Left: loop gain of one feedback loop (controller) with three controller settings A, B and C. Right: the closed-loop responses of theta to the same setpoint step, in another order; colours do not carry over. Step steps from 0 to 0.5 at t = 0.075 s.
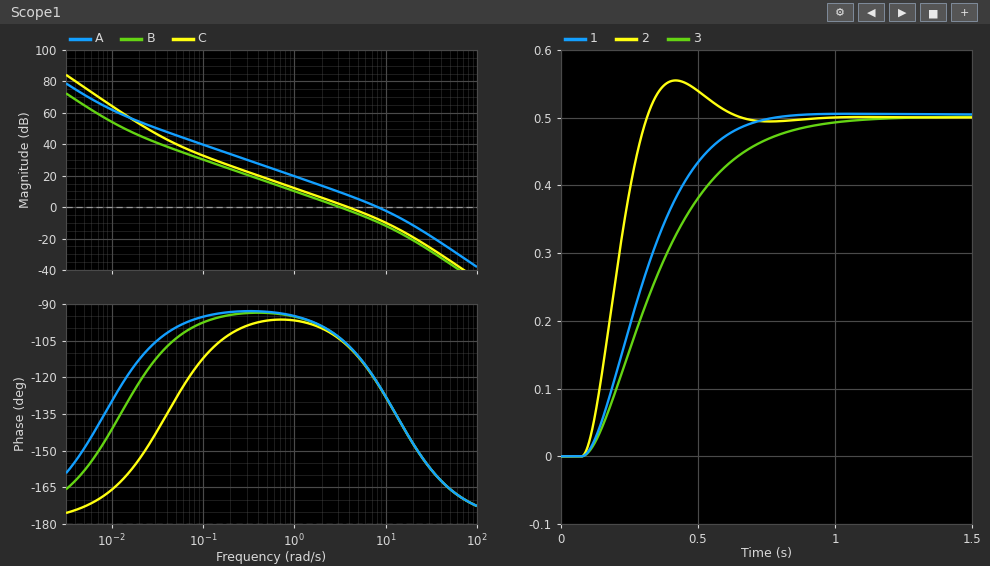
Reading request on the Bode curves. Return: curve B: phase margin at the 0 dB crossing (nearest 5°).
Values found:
75°
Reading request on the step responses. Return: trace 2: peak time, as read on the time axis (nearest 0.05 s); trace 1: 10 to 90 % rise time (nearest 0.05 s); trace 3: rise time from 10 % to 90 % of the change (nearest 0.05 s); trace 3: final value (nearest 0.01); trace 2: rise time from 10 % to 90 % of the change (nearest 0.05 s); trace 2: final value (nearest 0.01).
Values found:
0.40 s
0.40 s
0.50 s
0.50
0.15 s
0.50
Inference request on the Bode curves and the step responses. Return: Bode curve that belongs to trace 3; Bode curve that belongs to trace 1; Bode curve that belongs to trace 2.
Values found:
B
C
A
